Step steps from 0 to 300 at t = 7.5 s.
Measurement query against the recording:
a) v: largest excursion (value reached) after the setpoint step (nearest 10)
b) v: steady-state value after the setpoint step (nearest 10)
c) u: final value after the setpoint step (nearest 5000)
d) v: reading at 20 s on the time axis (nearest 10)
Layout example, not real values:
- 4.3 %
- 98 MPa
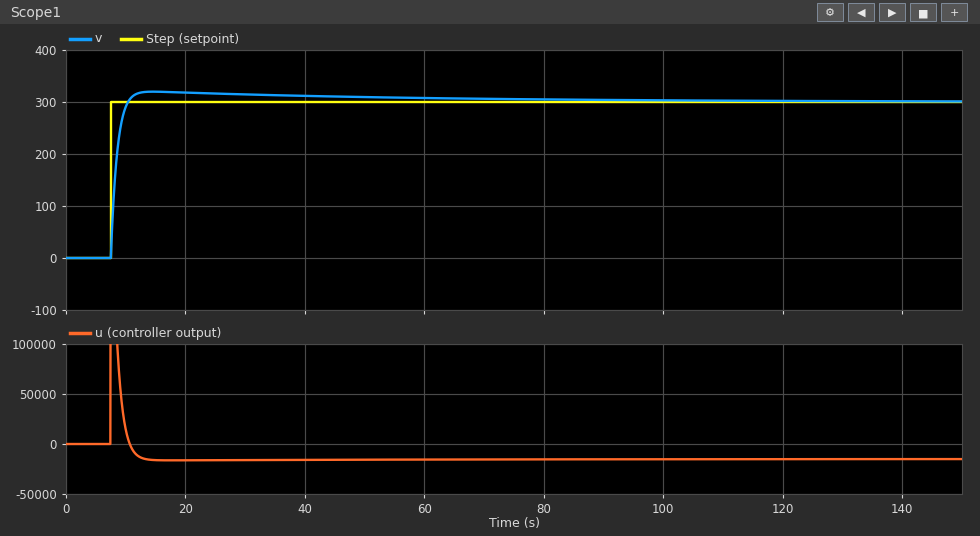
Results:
- 320
- 300
- -15000
- 320
